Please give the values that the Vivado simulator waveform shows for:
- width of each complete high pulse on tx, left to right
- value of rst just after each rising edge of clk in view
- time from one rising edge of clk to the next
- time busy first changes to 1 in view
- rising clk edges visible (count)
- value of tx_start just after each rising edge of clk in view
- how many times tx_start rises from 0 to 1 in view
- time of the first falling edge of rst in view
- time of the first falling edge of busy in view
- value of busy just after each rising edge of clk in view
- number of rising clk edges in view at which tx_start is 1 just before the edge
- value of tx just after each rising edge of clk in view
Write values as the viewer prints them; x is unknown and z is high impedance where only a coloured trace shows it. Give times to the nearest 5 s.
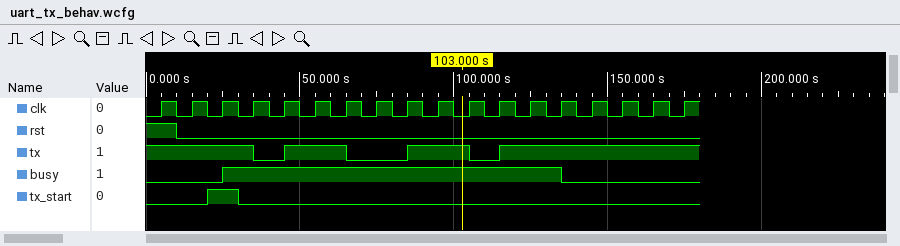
20 s, 20 s
1 0 0 0 0 0 0 0 0 0 0 0 0 0 0 0 0 0
10 s
25 s
18
0 0 1 0 0 0 0 0 0 0 0 0 0 0 0 0 0 0
1
10 s
135 s
0 0 1 1 1 1 1 1 1 1 1 1 1 0 0 0 0 0
1
1 1 1 0 1 1 0 0 1 1 0 1 1 1 1 1 1 1
